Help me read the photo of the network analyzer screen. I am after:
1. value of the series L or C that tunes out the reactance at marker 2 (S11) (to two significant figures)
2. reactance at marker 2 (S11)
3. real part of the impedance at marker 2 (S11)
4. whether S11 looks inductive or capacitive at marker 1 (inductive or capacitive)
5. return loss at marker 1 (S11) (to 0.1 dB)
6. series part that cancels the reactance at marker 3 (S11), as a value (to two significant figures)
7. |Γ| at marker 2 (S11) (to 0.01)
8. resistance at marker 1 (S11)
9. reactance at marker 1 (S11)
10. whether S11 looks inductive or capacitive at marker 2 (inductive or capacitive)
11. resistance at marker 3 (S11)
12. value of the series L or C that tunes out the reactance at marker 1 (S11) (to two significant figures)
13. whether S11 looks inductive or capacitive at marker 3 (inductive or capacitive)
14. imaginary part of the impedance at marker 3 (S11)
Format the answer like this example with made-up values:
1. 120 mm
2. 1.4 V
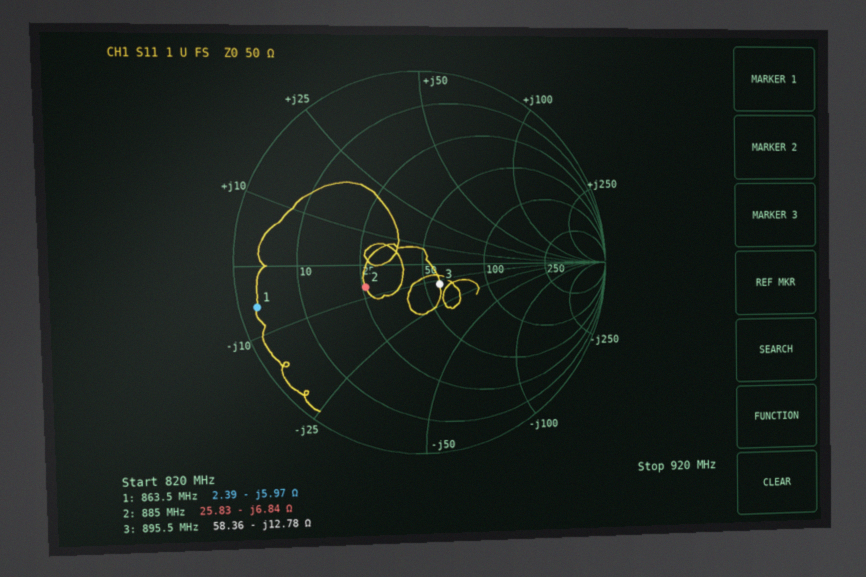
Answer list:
1. 1.2 nH
2. -6.84 Ω
3. 25.83 Ω
4. capacitive
5. 0.8 dB
6. 2.3 nH
7. 0.33
8. 2.39 Ω
9. -5.97 Ω
10. capacitive
11. 58.36 Ω
12. 1.1 nH
13. capacitive
14. -12.78 Ω
